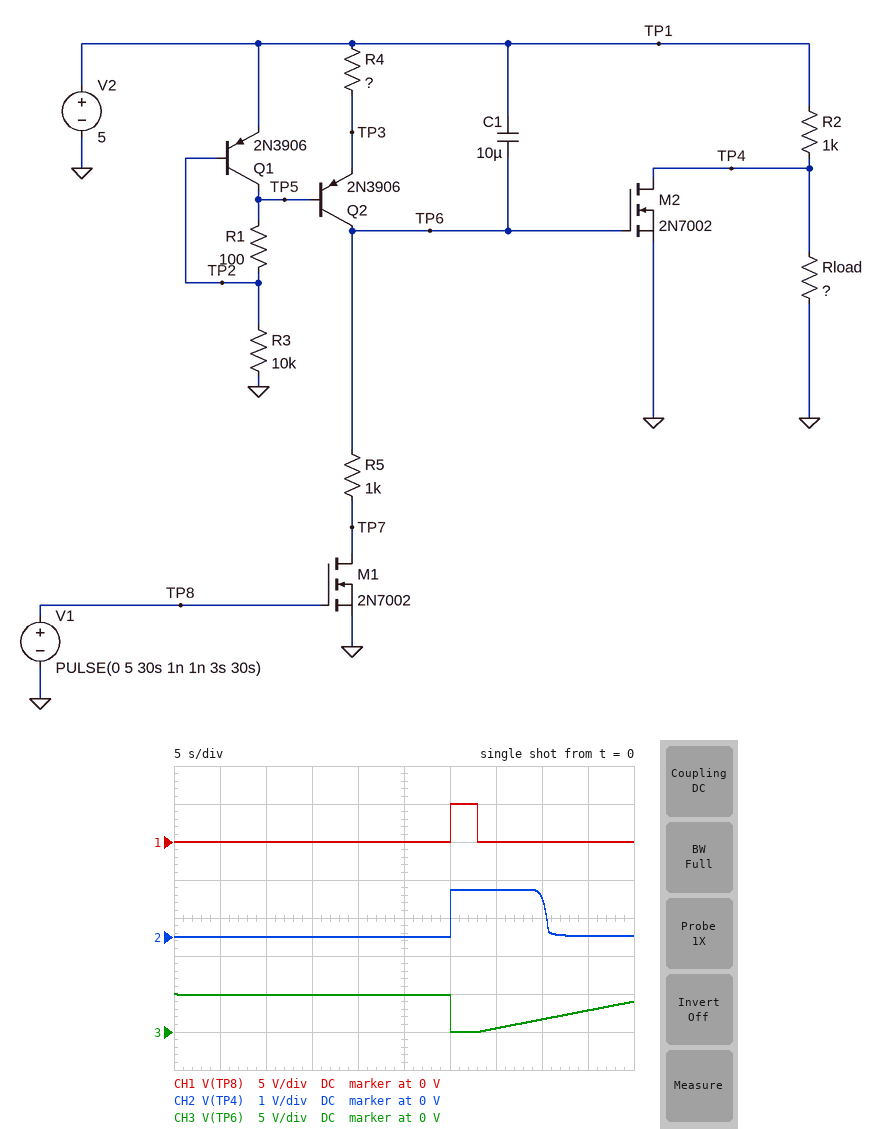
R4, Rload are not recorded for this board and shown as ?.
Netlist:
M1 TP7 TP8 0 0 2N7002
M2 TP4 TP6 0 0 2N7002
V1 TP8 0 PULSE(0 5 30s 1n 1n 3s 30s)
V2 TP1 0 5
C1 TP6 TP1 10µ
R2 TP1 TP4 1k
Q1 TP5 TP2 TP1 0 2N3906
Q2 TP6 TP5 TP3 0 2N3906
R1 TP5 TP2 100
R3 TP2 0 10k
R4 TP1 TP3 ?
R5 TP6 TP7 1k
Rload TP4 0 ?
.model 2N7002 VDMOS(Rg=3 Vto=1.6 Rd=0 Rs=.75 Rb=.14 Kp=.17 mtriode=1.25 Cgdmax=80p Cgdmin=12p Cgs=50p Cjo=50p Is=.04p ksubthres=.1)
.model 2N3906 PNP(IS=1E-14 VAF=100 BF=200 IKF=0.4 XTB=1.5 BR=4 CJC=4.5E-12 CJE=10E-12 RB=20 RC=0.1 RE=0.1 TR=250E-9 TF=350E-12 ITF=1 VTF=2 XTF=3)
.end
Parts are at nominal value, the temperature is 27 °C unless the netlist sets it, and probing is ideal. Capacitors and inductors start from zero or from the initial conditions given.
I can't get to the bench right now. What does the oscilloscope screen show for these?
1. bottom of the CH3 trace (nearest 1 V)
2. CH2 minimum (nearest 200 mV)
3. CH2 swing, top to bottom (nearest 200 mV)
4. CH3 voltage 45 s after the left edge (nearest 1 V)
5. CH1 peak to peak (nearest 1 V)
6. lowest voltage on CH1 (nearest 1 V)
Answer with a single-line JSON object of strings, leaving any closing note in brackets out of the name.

{"bottom of the CH3 trace": "0 V", "CH2 minimum": "0 V", "CH2 swing, top to bottom": "1.2 V", "CH3 voltage 45 s after the left edge": "3 V", "CH1 peak to peak": "5 V", "lowest voltage on CH1": "0 V"}
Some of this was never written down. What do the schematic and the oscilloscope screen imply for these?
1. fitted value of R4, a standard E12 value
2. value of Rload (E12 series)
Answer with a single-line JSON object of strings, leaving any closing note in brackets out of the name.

{"fitted value of R4, a standard E12 value": "39 kΩ", "value of Rload": "330 Ω"}
